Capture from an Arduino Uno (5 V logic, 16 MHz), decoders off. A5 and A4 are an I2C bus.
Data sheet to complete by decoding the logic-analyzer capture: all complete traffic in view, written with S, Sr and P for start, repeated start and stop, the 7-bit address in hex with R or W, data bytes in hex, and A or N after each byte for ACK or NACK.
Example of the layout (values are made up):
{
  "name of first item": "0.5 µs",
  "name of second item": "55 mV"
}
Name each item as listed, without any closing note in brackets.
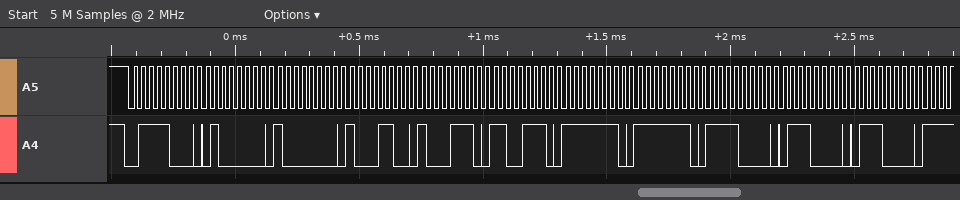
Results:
{
  "all complete traffic in view, written with S, Sr and P for start, repeated start and stop, the 7-bit address in hex with R or W, data bytes in hex, and A or N after each byte for ACK or NACK": "S 3CW A 40 A 80 A 8C A 8E A CE A FE A FE A F0 A 70 A 70 A"
}
